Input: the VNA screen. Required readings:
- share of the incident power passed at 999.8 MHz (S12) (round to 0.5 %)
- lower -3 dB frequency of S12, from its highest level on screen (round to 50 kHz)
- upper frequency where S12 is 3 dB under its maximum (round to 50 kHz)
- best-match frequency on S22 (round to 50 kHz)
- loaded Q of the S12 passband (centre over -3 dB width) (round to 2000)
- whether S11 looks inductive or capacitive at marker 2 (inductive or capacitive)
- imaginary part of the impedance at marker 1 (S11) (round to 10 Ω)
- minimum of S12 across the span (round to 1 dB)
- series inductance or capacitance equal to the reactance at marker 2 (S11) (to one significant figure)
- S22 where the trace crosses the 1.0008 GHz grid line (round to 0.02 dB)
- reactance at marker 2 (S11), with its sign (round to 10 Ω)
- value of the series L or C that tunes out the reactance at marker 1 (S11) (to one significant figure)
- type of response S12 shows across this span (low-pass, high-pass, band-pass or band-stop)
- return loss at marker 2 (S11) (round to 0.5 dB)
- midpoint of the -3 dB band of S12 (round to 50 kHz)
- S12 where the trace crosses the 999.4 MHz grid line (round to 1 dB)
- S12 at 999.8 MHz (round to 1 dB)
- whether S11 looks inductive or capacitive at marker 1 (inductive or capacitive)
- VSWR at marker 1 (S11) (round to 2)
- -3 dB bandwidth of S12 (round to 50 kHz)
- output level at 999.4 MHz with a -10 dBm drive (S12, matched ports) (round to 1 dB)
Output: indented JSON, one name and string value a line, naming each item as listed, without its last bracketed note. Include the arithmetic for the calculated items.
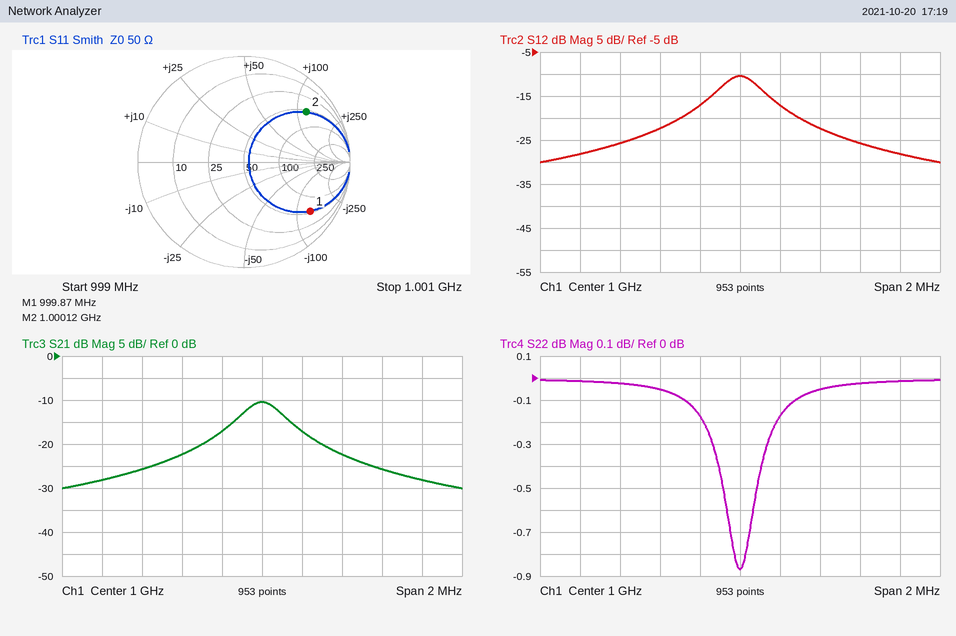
{
  "share of the incident power passed at 999.8 MHz (S12)": "10^(-17/10) ≈ 2.0 %",
  "lower -3 dB frequency of S12, from its highest level on screen": "999.90 MHz",
  "upper frequency where S12 is 3 dB under its maximum": "1.00010 GHz",
  "best-match frequency on S22": "1.00000 GHz",
  "loaded Q of the S12 passband (centre over -3 dB width)": "1 GHz / 200 kHz ≈ 5000, so 4000 to the nearest 2000",
  "whether S11 looks inductive or capacitive at marker 2": "inductive",
  "imaginary part of the impedance at marker 1 (S11)": "-130 Ω",
  "minimum of S12 across the span": "-30 dB",
  "series inductance or capacitance equal to the reactance at marker 2 (S11)": "L = 120 Ω/(2π × 1.00012 GHz) ≈ 19.1 nH, so 20 nH to one significant figure",
  "S22 where the trace crosses the 1.0008 GHz grid line": "-0.02 dB",
  "reactance at marker 2 (S11), with its sign": "+120 Ω",
  "value of the series L or C that tunes out the reactance at marker 1 (S11)": "L = 130 Ω/(2π × 999.87 MHz) ≈ 20.7 nH, so 20 nH to one significant figure",
  "type of response S12 shows across this span": "band-pass",
  "return loss at marker 2 (S11)": "2.5 dB",
  "midpoint of the -3 dB band of S12": "1.00000 GHz",
  "S12 where the trace crosses the 999.4 MHz grid line": "-26 dB",
  "S12 at 999.8 MHz": "-17 dB",
  "whether S11 looks inductive or capacitive at marker 1": "capacitive",
  "VSWR at marker 1 (S11)": "8",
  "-3 dB bandwidth of S12": "1.00010 GHz − 999.90 MHz = 200 kHz",
  "output level at 999.4 MHz with a -10 dBm drive (S12, matched ports)": "-10 dBm + (-26 dB) = -36 dBm"
}
